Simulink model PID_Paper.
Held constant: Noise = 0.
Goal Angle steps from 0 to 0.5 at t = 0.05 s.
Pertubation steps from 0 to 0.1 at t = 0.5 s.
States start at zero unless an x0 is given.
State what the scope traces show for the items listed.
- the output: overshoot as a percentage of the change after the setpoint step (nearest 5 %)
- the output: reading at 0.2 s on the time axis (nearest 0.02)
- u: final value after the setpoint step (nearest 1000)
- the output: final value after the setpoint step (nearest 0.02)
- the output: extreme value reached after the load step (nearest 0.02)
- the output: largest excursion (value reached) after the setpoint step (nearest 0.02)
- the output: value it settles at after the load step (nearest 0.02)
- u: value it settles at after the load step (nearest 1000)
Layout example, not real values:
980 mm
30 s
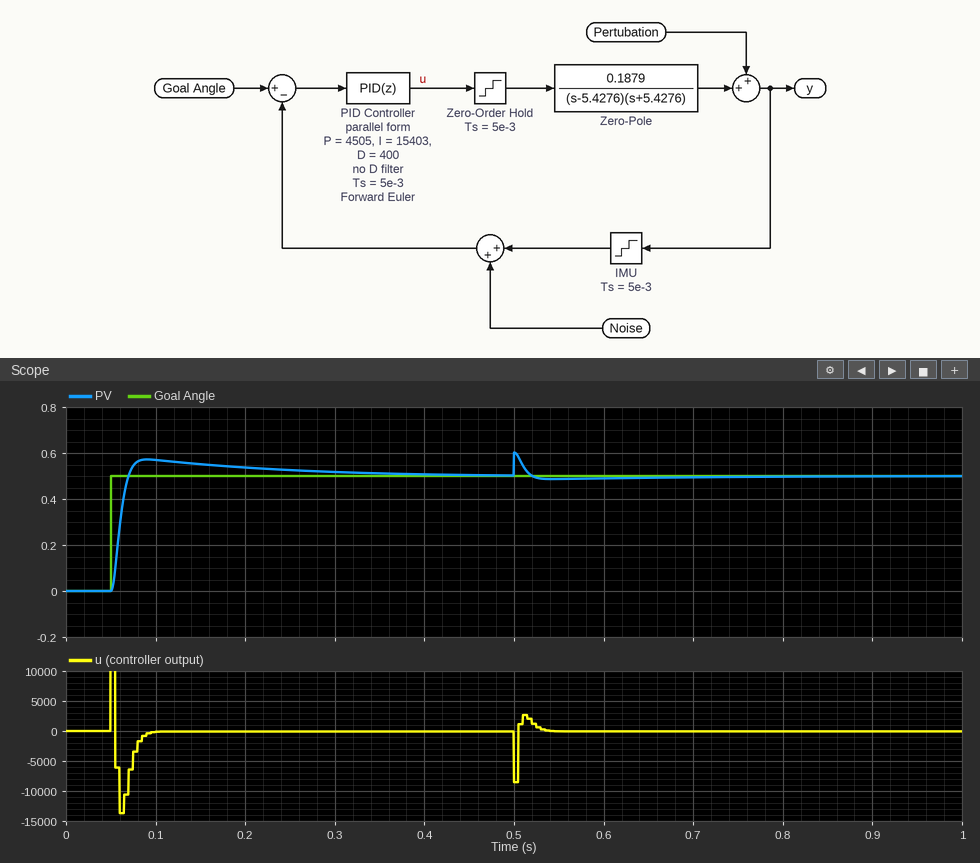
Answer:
15 %
0.54
0
0.50
0.60
0.58
0.50
0
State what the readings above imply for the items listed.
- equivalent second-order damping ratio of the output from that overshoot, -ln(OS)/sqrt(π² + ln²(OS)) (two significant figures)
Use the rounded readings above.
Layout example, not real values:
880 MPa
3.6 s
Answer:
0.52
